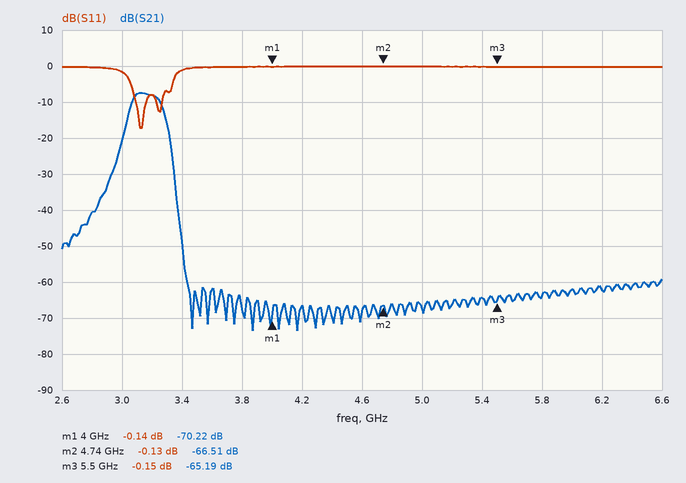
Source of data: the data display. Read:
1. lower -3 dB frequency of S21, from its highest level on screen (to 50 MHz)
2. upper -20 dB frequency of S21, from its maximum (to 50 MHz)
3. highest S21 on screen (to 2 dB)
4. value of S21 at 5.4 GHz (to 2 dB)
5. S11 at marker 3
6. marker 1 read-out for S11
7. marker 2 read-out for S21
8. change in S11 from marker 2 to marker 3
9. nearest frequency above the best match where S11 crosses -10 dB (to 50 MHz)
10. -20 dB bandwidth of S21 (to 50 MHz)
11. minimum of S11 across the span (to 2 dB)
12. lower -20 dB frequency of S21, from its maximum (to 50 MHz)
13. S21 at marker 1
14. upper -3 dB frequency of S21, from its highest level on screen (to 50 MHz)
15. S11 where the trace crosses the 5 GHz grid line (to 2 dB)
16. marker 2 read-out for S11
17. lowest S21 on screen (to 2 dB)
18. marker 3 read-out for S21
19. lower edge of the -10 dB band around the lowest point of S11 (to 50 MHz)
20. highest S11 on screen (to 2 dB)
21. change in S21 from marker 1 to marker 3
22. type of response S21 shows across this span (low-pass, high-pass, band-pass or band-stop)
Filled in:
3.05 GHz
3.35 GHz
-8 dB
-64 dB
-0.15 dB
-0.14 dB
-66.51 dB
-0.02 dB
3.15 GHz
400 MHz
-18 dB
2.95 GHz
-70.22 dB
3.25 GHz
0 dB
-0.13 dB
-74 dB
-65.19 dB
3.10 GHz
0 dB
5.03 dB
band-pass
